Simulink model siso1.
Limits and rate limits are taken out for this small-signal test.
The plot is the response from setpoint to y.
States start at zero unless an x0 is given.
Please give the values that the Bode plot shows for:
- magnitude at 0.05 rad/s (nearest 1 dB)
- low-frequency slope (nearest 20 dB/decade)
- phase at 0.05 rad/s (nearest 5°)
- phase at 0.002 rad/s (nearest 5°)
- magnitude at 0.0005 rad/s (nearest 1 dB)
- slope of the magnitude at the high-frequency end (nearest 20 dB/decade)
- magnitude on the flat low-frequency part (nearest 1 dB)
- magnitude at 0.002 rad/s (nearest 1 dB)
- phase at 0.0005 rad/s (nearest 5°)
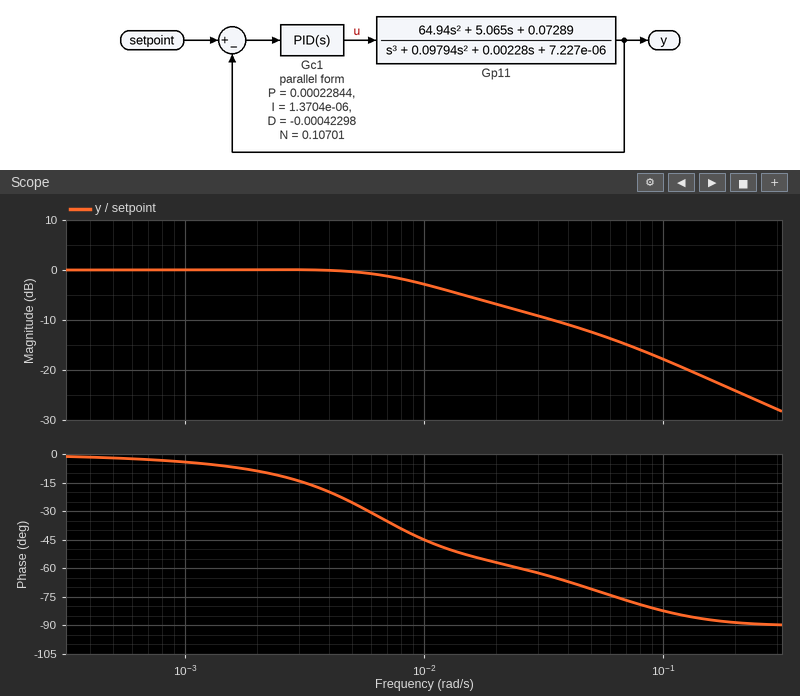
-12 dB
0 dB/decade
-70°
-10°
0 dB
-20 dB/decade
0 dB
0 dB
0°
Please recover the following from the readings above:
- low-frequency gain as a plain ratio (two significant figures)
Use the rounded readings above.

1.0
